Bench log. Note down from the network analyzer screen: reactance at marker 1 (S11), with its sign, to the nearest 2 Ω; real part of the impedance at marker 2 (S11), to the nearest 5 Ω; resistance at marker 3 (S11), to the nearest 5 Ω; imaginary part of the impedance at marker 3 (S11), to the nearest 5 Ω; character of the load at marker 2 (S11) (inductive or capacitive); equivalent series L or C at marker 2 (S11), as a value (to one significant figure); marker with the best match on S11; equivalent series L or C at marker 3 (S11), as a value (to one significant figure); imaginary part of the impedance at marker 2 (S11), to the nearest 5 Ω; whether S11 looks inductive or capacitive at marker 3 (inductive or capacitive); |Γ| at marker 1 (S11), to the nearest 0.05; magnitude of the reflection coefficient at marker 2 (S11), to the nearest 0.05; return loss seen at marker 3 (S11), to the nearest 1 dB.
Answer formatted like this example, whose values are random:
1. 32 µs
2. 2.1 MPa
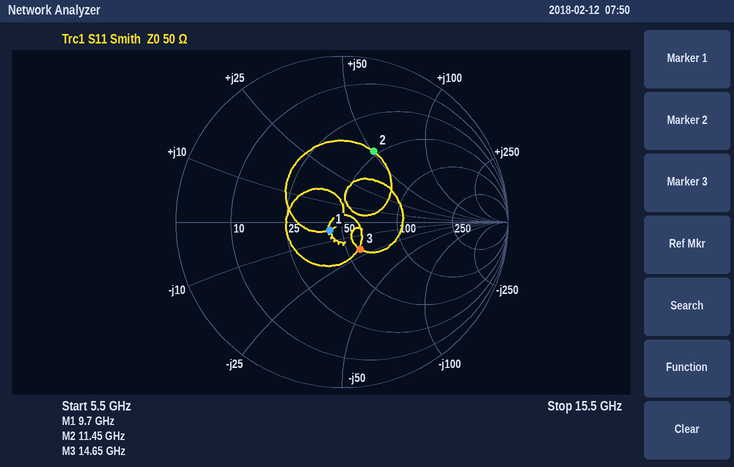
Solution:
1. -4 Ω
2. 45 Ω
3. 60 Ω
4. -20 Ω
5. inductive
6. 700 pH
7. marker 1
8. 500 fF
9. +50 Ω
10. capacitive
11. 0.10
12. 0.45
13. 14 dB
